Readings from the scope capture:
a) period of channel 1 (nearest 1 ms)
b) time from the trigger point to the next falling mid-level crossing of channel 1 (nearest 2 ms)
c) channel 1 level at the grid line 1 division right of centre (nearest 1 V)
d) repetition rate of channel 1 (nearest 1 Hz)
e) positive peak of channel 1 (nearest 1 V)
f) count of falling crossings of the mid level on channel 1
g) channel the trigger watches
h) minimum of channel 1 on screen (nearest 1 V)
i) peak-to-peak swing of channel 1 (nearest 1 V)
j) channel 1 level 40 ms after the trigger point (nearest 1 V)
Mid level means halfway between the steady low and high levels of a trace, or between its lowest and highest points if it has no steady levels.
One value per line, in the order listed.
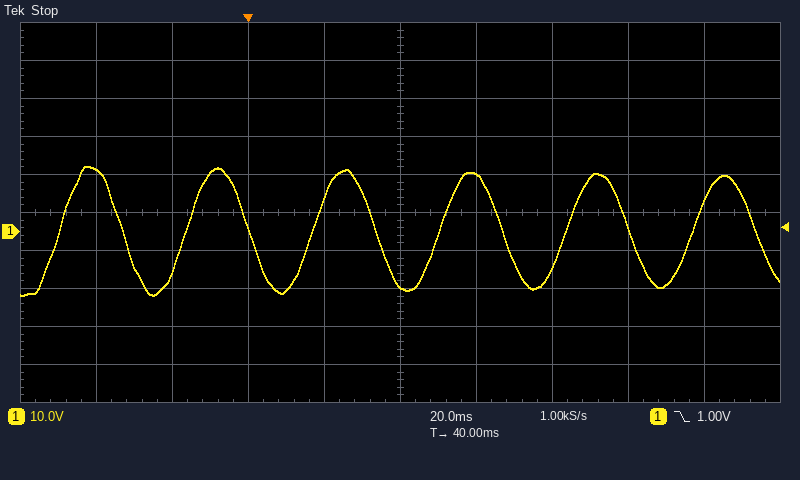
33 ms
34 ms
15 V
30 Hz
17 V
6
channel 1
-17 V
34 V
-14 V
